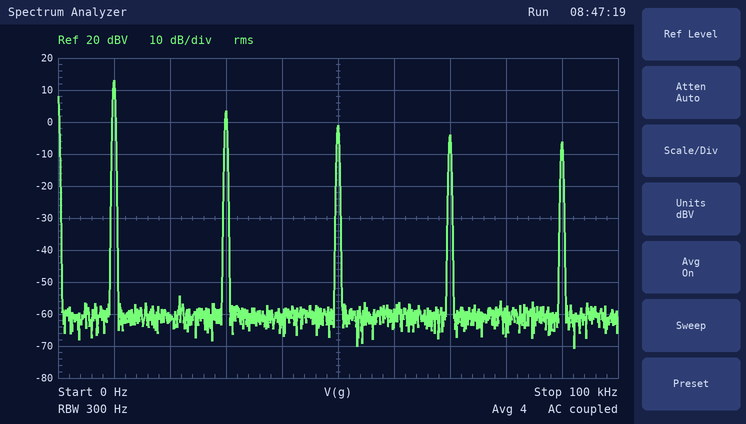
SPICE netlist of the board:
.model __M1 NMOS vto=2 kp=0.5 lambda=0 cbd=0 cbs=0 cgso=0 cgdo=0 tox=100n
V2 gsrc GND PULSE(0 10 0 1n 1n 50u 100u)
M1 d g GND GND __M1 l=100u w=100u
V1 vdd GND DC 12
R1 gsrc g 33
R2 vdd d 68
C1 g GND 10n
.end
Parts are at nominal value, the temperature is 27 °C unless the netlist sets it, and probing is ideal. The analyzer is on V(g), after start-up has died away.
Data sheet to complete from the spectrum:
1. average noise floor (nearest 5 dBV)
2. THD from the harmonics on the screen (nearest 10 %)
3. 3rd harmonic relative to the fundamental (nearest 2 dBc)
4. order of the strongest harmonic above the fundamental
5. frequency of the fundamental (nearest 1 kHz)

-60 dBV
40 %
-10 dBc
3
10 kHz
